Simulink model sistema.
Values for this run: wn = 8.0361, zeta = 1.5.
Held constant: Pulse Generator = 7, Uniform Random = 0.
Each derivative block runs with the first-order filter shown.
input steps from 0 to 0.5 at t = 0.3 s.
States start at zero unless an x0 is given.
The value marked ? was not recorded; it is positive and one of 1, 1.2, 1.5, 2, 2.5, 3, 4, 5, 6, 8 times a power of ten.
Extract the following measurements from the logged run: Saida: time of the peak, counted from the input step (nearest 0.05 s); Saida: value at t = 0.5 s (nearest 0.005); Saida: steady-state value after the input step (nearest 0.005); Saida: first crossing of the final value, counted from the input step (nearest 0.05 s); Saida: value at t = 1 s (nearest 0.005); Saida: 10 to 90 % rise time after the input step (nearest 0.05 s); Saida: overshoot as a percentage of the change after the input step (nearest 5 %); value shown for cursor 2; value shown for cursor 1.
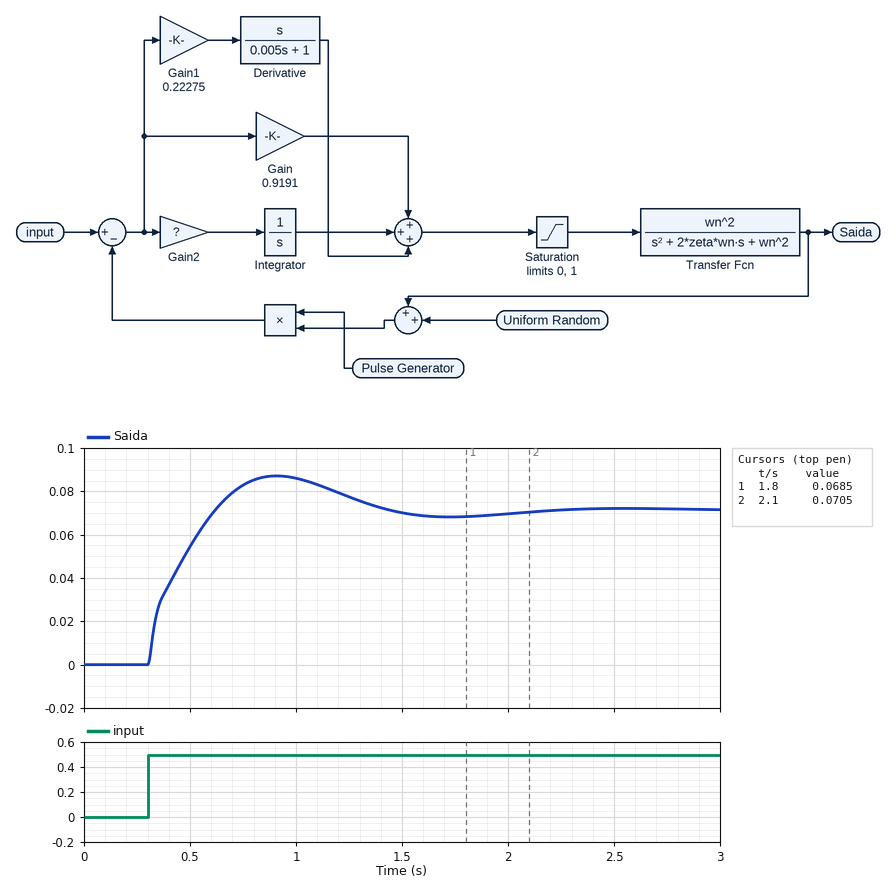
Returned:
0.60 s
0.055
0.070
0.30 s
0.085
0.25 s
20 %
0.0705
0.0685
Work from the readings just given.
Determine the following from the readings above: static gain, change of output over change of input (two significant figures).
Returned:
0.14
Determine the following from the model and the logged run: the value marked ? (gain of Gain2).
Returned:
5
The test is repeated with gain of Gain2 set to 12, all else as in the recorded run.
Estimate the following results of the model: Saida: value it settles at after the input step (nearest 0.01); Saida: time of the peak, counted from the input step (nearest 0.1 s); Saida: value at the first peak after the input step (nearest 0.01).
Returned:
0.07
0.4 s
0.10
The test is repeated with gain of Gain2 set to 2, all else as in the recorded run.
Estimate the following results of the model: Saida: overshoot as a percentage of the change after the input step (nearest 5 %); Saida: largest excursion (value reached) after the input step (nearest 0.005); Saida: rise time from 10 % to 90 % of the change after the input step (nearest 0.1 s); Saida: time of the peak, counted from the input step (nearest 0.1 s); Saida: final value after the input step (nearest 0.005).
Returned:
10 %
0.080
0.4 s
0.9 s
0.070
